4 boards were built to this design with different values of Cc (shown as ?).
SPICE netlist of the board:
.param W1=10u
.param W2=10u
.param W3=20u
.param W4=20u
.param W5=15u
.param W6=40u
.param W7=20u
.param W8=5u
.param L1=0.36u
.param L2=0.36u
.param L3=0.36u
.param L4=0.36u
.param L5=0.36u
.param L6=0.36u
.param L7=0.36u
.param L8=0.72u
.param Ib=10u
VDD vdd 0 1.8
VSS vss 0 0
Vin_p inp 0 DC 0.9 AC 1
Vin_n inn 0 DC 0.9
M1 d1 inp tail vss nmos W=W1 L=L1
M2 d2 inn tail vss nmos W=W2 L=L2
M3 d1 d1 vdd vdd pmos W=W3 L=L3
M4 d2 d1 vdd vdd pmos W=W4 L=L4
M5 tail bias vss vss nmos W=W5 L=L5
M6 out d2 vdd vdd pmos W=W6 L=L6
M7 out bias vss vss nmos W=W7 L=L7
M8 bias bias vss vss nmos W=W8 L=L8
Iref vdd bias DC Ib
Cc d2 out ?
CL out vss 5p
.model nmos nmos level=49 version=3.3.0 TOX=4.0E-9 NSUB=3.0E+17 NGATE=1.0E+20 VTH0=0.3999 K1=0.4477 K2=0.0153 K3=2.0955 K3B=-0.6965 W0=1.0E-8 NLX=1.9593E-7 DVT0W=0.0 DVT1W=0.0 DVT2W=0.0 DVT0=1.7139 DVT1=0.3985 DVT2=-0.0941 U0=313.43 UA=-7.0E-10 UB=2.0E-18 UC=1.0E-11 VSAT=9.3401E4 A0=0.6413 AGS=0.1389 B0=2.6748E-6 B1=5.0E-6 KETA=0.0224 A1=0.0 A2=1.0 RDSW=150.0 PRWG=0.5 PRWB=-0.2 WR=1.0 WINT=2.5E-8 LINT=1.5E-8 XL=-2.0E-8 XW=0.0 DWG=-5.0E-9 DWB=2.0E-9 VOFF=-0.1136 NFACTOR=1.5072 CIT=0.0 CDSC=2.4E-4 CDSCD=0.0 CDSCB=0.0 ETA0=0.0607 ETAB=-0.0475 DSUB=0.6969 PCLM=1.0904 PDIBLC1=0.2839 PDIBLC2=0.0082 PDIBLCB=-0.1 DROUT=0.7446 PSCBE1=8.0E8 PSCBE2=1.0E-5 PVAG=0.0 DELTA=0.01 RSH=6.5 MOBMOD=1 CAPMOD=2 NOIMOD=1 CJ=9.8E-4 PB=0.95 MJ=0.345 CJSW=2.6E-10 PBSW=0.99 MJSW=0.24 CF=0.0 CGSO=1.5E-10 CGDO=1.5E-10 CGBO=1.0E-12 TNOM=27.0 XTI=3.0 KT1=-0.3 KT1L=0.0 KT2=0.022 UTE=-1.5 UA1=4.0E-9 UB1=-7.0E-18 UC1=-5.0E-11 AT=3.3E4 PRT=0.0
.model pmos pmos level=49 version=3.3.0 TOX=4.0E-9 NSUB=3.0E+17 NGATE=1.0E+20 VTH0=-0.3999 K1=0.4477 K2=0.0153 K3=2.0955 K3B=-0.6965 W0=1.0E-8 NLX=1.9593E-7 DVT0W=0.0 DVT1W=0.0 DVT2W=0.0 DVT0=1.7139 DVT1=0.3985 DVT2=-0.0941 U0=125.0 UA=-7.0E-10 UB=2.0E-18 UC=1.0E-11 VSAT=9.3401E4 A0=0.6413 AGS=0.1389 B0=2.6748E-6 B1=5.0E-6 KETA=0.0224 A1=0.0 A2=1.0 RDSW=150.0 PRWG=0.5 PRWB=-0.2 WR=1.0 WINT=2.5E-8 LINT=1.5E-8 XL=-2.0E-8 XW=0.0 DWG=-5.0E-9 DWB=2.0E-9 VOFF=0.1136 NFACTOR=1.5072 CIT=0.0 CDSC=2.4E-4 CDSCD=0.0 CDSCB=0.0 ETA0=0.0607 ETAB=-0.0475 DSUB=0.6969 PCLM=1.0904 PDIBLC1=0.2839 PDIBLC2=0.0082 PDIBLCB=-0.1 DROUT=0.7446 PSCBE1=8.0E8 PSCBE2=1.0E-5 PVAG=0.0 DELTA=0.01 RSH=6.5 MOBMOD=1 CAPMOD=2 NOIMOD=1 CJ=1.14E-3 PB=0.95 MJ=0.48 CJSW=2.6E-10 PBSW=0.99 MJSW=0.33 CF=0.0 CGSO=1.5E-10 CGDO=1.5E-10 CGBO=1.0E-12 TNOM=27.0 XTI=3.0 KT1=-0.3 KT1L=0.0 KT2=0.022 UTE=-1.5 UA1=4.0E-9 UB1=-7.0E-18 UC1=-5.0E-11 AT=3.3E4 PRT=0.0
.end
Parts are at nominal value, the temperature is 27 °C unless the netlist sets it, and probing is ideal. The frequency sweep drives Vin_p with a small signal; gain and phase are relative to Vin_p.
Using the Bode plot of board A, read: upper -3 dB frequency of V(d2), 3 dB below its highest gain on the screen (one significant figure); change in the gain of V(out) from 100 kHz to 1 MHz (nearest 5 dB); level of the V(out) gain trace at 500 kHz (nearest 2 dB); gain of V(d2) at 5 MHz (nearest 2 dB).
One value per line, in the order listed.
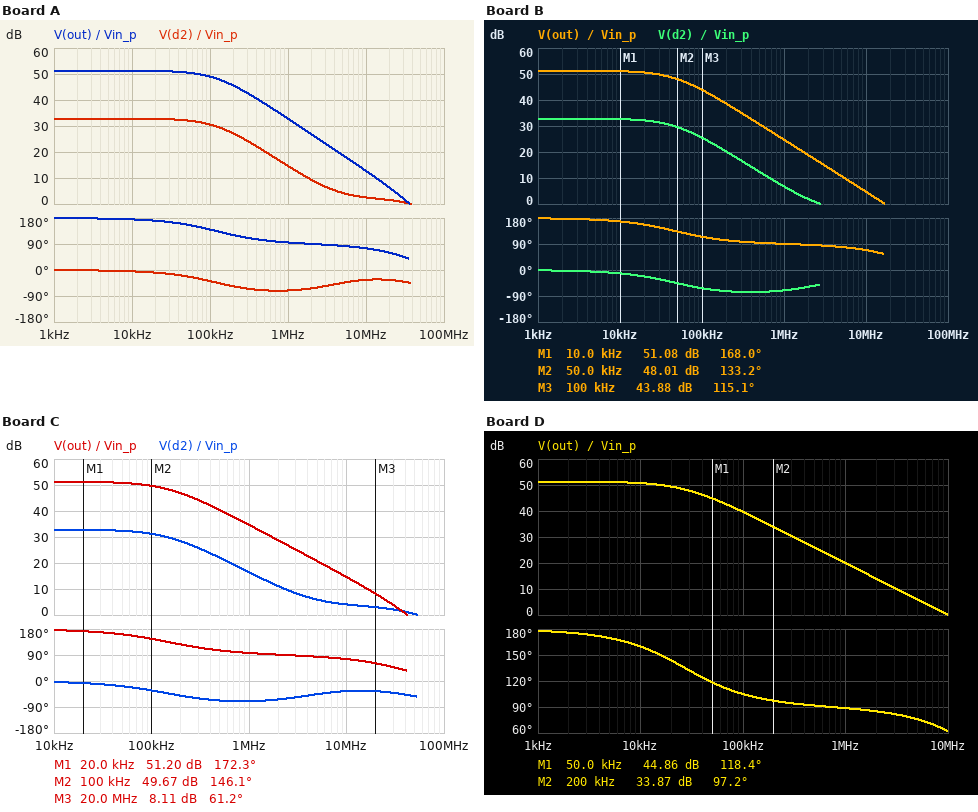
100 kHz
-15 dB
38 dB
4 dB
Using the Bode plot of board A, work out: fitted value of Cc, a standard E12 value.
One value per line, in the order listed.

1.5 pF
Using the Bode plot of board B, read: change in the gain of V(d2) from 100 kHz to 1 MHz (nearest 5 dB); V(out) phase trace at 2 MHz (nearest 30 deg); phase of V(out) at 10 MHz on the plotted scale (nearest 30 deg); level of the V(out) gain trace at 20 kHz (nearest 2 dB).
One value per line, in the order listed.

-20 dB
90 deg
60 deg
50 dB
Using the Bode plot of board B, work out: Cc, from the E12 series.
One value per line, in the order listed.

3.9 pF
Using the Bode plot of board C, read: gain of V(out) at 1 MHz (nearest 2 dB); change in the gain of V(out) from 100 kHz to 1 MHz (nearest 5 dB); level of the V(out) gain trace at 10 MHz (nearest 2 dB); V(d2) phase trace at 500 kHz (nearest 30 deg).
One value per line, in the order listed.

34 dB
-15 dB
14 dB
-60 deg
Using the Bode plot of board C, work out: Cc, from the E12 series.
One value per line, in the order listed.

1.2 pF
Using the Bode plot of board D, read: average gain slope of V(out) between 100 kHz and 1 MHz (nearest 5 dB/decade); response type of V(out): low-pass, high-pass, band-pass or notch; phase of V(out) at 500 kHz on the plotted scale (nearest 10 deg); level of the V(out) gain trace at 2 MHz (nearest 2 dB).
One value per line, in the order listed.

-20 dB/decade
low-pass
90 deg
14 dB
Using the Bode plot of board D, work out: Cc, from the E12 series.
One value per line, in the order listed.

6.8 pF
